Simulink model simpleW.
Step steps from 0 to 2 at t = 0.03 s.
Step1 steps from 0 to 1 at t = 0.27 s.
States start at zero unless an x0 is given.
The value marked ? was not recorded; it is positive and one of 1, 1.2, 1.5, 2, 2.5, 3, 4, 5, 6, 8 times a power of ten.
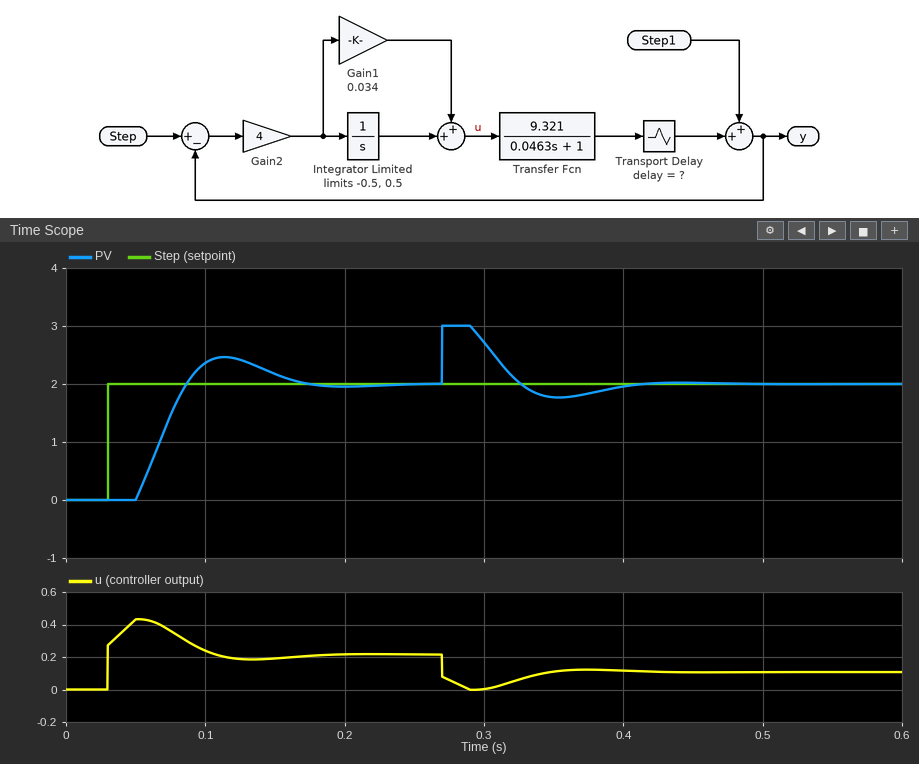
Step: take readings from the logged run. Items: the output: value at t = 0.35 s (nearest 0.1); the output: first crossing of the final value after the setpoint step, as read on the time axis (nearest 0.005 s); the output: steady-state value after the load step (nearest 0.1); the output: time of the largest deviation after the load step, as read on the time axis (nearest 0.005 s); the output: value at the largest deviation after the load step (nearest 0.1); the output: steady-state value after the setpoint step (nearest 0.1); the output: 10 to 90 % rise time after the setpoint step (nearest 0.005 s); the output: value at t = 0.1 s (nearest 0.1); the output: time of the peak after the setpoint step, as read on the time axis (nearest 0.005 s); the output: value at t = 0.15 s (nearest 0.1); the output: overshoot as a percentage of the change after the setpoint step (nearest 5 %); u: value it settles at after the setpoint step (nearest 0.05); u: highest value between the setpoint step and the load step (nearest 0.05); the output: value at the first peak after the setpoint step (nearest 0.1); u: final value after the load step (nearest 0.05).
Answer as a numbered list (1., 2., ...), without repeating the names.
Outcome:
1. 1.8
2. 0.085 s
3. 2.0
4. 0.280 s
5. 3.0
6. 2.0
7. 0.030 s
8. 2.4
9. 0.115 s
10. 2.2
11. 25 %
12. 0.20
13. 0.45
14. 2.5
15. 0.10
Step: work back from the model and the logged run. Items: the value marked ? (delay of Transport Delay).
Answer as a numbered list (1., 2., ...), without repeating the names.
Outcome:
1. 0.02
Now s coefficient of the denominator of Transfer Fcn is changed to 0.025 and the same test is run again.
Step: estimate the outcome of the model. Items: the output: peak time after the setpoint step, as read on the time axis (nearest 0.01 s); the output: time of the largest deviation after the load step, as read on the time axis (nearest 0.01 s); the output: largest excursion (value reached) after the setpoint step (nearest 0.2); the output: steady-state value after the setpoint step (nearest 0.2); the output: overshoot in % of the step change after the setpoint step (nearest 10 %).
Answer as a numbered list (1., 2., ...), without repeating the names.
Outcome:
1. 0.09 s
2. 0.27 s
3. 2.6
4. 2.0
5. 30 %
